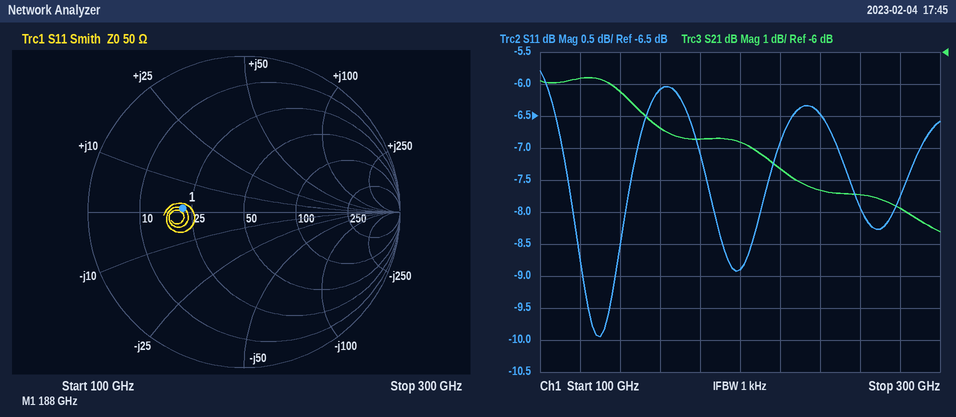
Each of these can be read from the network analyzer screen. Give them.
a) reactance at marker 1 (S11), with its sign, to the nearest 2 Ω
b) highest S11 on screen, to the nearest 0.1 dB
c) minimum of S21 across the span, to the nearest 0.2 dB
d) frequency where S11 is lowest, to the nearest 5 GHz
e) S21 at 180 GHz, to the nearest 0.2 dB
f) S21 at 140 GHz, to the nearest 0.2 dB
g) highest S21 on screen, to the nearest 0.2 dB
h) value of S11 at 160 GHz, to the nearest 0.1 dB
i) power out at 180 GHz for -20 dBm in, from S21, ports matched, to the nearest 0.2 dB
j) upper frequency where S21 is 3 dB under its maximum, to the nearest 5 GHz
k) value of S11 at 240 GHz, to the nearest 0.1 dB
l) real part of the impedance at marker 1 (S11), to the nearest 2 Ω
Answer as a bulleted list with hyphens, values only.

- +2 Ω
- -5.8 dB
- -11.6 dB
- 130 GHz
- -8.8 dB
- -7.2 dB
- -6.8 dB
- -6.1 dB
- -28.8 dBm
- 225 GHz
- -6.5 dB
- 22 Ω
